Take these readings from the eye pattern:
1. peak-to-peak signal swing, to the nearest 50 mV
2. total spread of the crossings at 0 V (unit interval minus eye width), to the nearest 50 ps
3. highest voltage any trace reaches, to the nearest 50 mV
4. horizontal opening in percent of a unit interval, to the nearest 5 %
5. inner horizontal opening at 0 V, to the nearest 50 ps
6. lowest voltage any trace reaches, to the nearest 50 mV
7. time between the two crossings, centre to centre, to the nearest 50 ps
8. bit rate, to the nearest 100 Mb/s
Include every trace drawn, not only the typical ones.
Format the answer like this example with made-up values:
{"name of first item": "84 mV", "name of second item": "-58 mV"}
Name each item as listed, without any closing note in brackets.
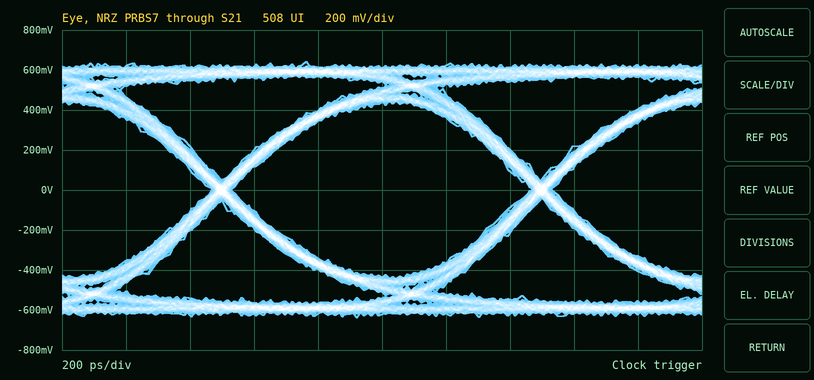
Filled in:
{"peak-to-peak signal swing, to the nearest 50 mV": "1.30 V", "total spread of the crossings at 0 V (unit interval minus eye width), to the nearest 50 ps": "50 ps", "highest voltage any trace reaches, to the nearest 50 mV": "650 mV", "horizontal opening in percent of a unit interval, to the nearest 5 %": "95 %", "inner horizontal opening at 0 V, to the nearest 50 ps": "950 ps", "lowest voltage any trace reaches, to the nearest 50 mV": "-650 mV", "time between the two crossings, centre to centre, to the nearest 50 ps": "1.00 ns", "bit rate, to the nearest 100 Mb/s": "1.0 Gb/s"}
